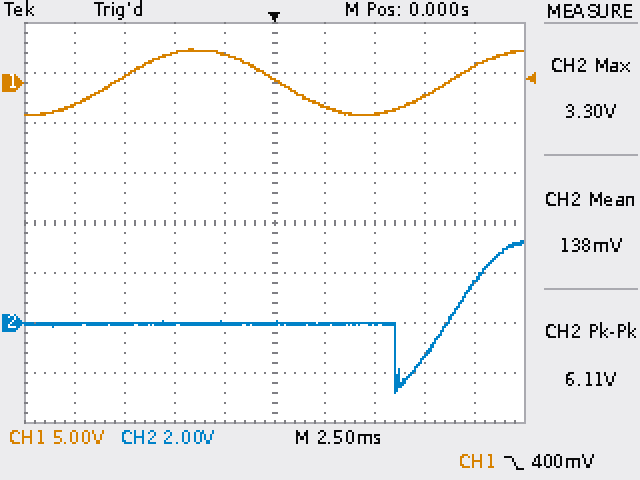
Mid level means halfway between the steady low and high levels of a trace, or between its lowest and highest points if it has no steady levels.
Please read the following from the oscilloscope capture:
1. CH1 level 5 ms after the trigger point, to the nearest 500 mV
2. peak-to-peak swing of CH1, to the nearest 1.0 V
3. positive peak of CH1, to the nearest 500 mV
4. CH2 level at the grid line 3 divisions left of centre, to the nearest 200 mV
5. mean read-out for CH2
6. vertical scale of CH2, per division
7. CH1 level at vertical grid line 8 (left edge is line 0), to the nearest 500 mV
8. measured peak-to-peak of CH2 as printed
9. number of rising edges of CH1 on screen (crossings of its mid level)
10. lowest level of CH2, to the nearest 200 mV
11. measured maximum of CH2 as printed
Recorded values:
-3.0 V
7.0 V
3.5 V
0.0 V
138 mV
2 V
-1.5 V
6.11 V
2
-2.8 V
3.30 V
